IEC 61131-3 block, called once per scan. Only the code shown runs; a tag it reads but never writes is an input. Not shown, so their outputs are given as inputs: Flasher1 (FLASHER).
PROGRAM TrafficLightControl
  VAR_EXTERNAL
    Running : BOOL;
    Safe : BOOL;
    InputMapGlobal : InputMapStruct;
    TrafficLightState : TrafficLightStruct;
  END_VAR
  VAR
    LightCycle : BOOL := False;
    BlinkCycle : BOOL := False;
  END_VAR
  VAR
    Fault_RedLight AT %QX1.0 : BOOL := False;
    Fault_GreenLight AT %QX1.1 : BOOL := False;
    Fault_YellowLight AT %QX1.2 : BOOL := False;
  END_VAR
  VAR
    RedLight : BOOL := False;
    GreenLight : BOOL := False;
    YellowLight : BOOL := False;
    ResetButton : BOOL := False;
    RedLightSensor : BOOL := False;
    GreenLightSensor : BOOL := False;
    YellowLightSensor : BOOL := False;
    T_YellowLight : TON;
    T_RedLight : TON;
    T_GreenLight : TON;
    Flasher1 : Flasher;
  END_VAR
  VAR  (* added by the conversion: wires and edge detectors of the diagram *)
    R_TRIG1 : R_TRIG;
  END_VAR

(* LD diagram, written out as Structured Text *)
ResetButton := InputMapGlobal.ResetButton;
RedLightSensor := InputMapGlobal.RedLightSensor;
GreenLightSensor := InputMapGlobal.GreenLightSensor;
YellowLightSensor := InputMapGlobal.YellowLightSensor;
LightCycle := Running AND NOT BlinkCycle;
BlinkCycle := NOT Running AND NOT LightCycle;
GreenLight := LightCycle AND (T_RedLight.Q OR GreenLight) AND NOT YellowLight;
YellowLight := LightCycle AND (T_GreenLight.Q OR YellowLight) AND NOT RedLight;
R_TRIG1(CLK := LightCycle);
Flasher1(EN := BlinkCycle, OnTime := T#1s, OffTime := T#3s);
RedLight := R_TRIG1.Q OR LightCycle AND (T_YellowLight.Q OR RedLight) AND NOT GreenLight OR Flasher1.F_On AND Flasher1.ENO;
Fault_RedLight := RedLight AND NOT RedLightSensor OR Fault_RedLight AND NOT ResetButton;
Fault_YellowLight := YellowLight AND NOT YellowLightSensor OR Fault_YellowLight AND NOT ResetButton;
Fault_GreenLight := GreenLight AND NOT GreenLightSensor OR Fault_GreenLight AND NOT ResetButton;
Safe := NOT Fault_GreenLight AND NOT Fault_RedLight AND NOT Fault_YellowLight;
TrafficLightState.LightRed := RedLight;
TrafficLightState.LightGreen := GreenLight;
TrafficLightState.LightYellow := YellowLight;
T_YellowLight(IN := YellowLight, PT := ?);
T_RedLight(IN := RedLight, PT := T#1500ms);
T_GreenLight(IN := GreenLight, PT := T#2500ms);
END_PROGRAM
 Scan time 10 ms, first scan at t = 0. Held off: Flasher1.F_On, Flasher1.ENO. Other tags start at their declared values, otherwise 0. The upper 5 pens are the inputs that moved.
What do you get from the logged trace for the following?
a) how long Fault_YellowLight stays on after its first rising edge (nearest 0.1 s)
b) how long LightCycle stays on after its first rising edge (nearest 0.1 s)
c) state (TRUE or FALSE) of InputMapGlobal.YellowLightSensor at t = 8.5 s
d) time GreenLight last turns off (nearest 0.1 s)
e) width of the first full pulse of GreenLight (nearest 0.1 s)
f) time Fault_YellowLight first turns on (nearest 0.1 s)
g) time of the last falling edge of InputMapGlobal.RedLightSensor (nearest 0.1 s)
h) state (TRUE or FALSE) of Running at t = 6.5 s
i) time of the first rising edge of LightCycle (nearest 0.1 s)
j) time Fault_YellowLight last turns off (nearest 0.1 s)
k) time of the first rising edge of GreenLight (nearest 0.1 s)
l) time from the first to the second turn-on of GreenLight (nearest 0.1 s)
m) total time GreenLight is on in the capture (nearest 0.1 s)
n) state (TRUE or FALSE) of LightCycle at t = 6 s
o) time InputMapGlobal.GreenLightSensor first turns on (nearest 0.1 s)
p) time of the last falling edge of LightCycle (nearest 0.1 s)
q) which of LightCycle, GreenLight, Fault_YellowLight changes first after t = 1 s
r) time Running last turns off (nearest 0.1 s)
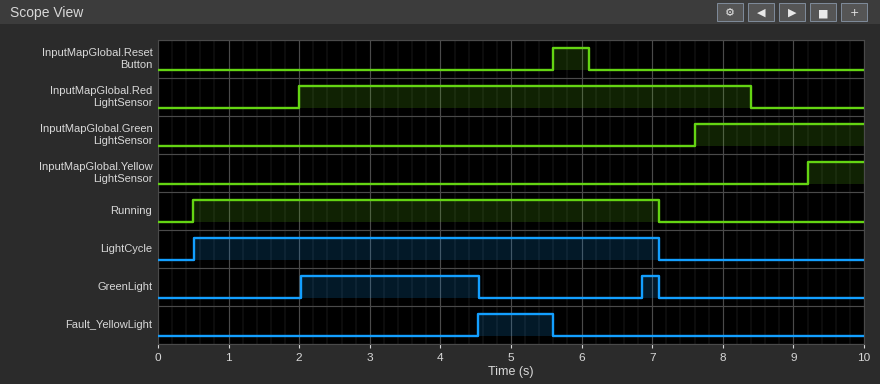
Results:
1.1 s
6.6 s
FALSE
7.1 s
2.5 s
4.5 s
8.4 s
TRUE
0.5 s
5.6 s
2.0 s
4.8 s
2.8 s
TRUE
7.6 s
7.1 s
GreenLight
7.1 s
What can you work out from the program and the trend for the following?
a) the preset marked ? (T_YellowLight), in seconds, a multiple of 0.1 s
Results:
0.8 s
